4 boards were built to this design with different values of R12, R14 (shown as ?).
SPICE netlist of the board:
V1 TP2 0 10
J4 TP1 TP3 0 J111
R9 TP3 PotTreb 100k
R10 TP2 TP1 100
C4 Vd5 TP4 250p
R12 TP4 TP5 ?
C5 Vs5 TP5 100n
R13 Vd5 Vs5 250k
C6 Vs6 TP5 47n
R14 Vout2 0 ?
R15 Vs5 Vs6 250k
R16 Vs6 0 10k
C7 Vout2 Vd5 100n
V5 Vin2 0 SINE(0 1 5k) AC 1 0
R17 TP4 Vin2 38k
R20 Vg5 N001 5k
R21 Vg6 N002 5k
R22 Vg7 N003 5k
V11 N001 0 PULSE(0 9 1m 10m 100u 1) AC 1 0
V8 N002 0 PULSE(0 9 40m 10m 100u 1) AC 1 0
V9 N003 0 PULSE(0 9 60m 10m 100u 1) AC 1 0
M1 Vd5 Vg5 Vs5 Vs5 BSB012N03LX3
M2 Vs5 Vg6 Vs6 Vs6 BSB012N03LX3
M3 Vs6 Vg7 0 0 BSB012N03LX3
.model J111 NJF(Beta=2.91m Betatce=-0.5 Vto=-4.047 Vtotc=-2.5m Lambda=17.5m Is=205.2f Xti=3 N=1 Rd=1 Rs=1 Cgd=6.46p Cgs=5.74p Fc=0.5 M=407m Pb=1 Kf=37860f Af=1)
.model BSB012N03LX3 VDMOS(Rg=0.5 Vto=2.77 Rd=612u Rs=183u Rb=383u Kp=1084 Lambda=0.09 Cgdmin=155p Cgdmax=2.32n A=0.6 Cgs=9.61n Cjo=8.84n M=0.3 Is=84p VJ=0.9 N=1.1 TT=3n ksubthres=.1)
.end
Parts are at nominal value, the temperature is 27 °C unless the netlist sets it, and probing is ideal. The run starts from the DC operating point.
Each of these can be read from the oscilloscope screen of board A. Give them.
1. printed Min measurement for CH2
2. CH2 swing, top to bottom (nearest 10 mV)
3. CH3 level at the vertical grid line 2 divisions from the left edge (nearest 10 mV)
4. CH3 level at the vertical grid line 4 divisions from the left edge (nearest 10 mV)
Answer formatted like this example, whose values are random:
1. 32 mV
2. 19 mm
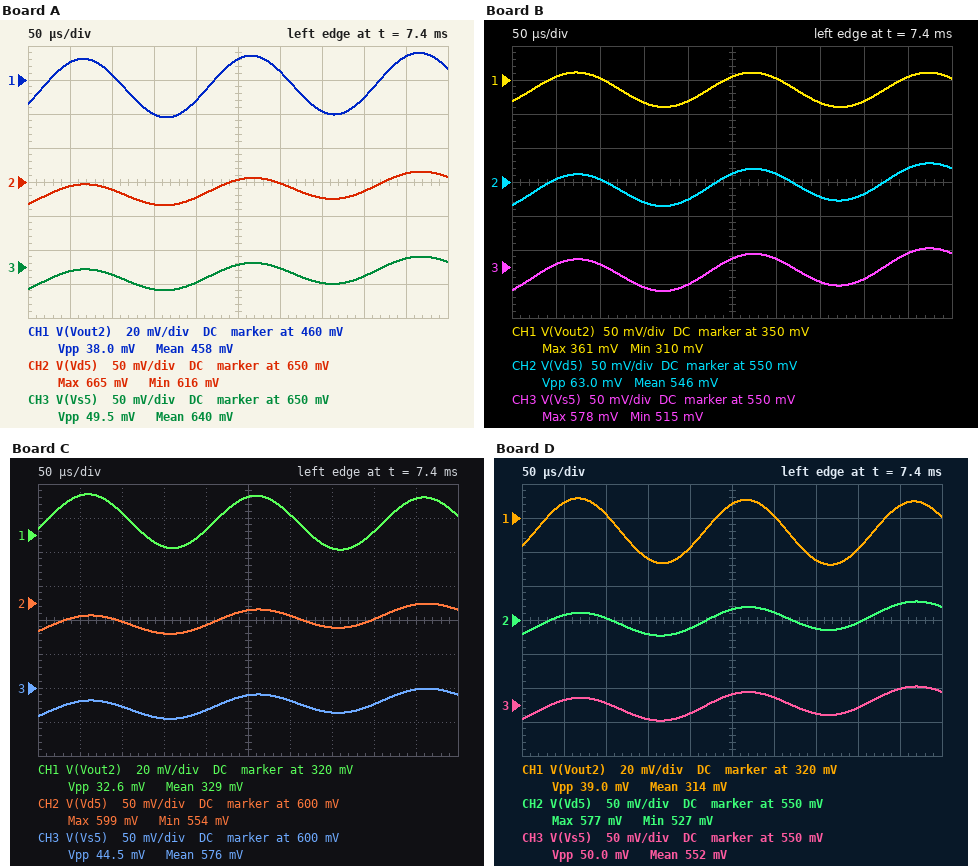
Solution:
1. 616 mV
2. 50 mV
3. 640 mV
4. 630 mV
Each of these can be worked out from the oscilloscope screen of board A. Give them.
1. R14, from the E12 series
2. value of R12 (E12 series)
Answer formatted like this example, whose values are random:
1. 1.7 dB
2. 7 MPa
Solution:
1. 120 kΩ
2. 82 kΩ
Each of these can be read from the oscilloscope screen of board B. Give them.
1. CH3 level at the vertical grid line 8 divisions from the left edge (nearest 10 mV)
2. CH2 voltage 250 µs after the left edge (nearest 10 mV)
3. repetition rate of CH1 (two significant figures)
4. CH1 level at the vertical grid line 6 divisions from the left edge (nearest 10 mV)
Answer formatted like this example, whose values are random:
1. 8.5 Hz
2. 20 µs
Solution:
1. 530 mV
2. 560 mV
3. 5.0 kHz
4. 350 mV
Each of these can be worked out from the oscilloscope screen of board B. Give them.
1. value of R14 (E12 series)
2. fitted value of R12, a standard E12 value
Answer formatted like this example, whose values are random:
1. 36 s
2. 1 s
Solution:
1. 82 kΩ
2. 33 kΩ
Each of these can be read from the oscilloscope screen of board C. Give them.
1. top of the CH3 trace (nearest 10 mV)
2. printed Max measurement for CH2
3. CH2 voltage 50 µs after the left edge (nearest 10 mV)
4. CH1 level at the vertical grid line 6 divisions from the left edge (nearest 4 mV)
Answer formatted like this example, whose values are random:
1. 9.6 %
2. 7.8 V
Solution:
1. 600 mV
2. 599 mV
3. 580 mV
4. 332 mV
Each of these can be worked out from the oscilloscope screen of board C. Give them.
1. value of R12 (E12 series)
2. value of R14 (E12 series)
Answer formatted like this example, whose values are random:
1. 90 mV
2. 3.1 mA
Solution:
1. 120 kΩ
2. 68 kΩ
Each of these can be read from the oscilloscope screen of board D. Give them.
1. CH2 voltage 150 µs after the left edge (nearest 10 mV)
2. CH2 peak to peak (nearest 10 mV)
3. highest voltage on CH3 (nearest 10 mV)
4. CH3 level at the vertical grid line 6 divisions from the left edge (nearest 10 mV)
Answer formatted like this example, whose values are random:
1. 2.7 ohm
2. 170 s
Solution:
1. 530 mV
2. 50 mV
3. 580 mV
4. 560 mV
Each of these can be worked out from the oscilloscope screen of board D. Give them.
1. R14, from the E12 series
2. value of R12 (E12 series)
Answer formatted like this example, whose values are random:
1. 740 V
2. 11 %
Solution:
1. 68 kΩ
2. 68 kΩ
